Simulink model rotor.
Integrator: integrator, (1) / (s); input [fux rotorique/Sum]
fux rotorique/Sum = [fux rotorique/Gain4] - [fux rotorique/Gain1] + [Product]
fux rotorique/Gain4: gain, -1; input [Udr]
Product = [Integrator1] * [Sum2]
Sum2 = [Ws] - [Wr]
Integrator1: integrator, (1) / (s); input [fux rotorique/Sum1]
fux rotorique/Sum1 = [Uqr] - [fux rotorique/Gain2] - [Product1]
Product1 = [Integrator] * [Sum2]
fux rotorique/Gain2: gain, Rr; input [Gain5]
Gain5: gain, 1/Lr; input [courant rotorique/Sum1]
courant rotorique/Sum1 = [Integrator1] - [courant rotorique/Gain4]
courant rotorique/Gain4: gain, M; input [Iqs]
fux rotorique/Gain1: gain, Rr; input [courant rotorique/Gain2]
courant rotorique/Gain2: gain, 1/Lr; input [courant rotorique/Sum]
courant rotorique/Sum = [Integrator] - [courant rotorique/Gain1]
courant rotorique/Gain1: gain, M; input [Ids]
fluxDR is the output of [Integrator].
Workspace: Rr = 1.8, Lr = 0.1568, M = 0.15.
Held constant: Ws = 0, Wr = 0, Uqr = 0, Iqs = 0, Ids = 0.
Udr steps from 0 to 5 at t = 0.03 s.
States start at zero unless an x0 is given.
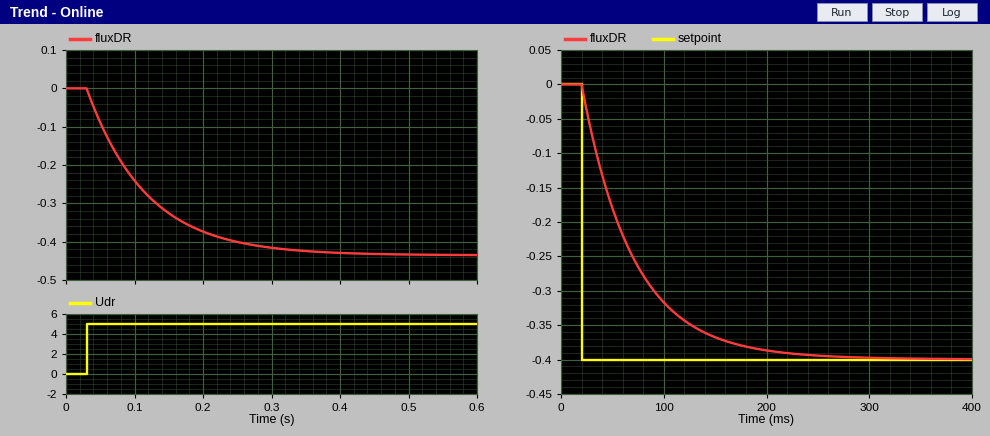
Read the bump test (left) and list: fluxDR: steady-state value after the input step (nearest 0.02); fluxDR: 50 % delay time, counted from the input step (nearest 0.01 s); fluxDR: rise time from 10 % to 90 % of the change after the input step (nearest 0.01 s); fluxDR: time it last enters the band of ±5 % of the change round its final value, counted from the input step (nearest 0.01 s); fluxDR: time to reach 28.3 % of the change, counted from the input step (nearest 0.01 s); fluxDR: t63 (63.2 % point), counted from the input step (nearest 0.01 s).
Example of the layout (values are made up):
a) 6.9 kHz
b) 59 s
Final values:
a) -0.44
b) 0.06 s
c) 0.19 s
d) 0.26 s
e) 0.03 s
f) 0.09 s
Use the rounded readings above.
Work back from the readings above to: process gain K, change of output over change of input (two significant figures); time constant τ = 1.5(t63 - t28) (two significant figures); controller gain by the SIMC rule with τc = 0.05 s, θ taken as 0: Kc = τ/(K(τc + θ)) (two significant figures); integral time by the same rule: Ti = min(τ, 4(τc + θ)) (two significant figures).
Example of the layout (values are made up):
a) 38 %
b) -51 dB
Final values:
a) -0.088
b) 0.090 s
c) -20
d) 0.090 s
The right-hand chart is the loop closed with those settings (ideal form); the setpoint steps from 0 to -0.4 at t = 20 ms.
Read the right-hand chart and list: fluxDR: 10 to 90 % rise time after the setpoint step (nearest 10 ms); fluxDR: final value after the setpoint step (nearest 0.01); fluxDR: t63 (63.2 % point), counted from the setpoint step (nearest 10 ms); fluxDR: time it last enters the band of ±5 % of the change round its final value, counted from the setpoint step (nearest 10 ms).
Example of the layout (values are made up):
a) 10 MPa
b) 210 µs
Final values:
a) 110 ms
b) -0.40
c) 50 ms
d) 160 ms
